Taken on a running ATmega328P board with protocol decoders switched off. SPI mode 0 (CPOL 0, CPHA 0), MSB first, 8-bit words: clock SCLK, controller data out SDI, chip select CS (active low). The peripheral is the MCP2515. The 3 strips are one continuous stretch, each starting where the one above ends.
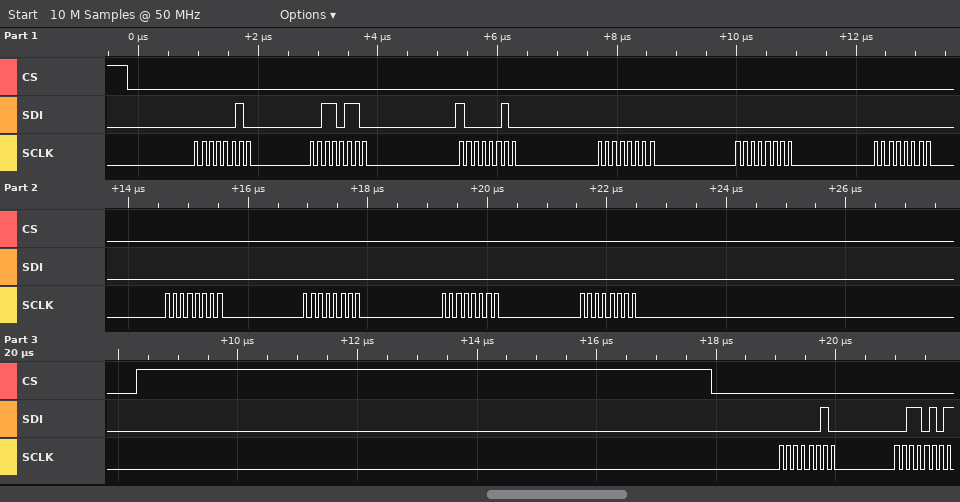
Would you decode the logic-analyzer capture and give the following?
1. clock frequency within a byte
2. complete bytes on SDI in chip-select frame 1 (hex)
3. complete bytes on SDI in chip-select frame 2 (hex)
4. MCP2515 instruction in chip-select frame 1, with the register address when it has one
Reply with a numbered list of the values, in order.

1. 8 MHz
2. 0x02 0x36 0x82 0x00 0x00 0x00 0x00 0x00 0x00 0x00
3. 0x02 0x35
4. WRITE 0x36
